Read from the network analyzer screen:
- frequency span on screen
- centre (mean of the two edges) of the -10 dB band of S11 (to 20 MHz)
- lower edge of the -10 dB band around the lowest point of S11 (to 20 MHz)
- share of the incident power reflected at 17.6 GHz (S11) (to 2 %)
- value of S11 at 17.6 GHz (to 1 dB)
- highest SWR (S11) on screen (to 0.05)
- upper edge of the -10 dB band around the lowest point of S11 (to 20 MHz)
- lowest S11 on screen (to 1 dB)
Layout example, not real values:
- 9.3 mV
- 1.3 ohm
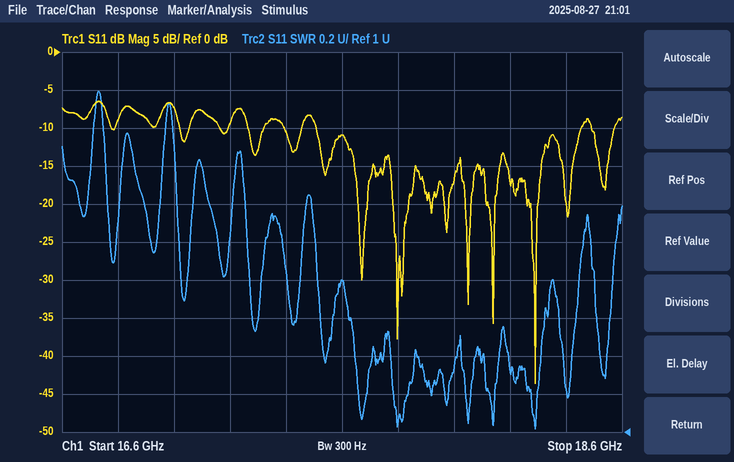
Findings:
- 2 GHz
- 17.98 GHz
- 17.50 GHz
- 8 %
- -11 dB
- 2.80
- 18.46 GHz
- -44 dB
